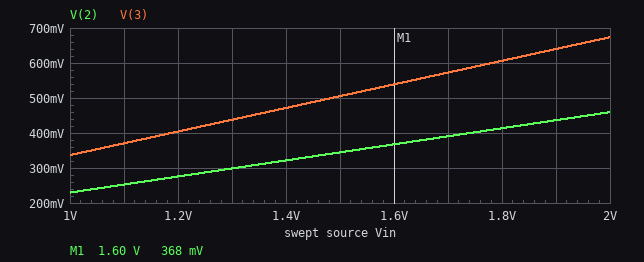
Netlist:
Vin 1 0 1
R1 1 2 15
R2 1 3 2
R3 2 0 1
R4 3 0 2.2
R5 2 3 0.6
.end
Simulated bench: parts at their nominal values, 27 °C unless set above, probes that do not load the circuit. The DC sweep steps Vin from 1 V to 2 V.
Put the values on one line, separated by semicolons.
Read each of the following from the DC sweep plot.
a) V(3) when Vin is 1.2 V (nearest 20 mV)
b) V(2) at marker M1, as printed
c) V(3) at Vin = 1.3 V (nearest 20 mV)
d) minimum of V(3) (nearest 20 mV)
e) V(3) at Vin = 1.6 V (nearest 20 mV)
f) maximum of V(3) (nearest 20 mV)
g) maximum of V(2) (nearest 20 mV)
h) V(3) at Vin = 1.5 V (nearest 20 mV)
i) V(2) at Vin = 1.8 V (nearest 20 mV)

400 mV; 368 mV; 440 mV; 340 mV; 540 mV; 680 mV; 460 mV; 500 mV; 420 mV
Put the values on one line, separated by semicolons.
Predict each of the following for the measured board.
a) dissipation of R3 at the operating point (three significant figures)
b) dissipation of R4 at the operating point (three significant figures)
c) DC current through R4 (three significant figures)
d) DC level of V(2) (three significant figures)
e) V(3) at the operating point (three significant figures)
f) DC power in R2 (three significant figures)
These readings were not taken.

52.8 mW; 51.6 mW; 153 mA; 230 mV; 337 mV; 220 mW
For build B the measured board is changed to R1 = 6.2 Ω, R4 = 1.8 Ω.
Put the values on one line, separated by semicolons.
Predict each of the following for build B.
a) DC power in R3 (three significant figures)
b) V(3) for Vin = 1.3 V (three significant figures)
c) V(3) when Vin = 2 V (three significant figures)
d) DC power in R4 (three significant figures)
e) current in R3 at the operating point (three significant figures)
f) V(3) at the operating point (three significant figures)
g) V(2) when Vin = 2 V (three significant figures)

66.9 mW; 445 mV; 684 mV; 65.0 mW; 259 mA; 342 mV; 517 mV
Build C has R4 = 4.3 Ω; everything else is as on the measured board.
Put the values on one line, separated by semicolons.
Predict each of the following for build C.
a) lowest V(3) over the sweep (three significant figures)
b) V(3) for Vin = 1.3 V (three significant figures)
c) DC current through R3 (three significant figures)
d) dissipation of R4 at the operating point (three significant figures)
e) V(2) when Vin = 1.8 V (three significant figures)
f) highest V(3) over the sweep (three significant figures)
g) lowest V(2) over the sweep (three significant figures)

391 mV; 508 mV; 263 mA; 35.5 mW; 473 mV; 782 mV; 263 mV
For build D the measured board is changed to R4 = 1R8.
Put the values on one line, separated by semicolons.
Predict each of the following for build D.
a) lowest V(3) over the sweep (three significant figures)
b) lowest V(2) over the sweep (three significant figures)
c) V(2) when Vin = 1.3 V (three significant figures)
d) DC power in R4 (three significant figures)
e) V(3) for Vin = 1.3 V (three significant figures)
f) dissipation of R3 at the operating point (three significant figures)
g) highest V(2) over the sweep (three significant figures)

317 mV; 218 mV; 283 mV; 55.8 mW; 412 mV; 47.4 mW; 435 mV
